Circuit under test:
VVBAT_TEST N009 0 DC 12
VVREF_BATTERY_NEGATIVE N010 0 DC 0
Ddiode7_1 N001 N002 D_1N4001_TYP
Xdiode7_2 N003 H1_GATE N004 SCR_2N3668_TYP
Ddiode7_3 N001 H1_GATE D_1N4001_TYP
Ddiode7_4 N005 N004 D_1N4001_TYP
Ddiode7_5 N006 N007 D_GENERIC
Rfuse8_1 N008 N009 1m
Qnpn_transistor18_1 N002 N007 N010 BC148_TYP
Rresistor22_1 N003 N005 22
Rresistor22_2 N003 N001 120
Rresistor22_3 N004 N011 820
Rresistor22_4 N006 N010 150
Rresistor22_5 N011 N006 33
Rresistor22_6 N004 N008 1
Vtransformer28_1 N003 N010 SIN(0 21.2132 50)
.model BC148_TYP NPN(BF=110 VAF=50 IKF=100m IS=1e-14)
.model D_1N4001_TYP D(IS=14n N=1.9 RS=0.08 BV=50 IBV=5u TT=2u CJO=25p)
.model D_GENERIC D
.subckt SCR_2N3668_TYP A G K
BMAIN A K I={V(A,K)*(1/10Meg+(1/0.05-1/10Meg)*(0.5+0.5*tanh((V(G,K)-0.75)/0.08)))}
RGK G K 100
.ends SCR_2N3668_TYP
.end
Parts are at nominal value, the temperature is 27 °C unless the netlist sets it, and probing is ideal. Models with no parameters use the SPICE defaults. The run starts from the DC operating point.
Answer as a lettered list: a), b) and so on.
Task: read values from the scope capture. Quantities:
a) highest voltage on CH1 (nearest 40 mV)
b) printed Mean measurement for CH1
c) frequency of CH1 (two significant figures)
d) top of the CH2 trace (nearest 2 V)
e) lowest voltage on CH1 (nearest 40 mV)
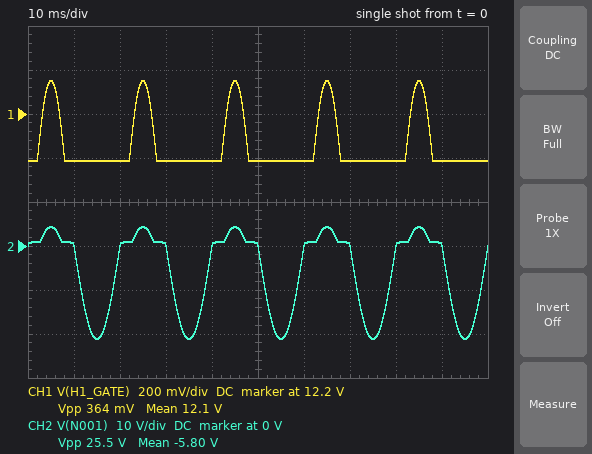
a) 12.36 V
b) 12.1 V
c) 50 Hz
d) 4 V
e) 12.00 V
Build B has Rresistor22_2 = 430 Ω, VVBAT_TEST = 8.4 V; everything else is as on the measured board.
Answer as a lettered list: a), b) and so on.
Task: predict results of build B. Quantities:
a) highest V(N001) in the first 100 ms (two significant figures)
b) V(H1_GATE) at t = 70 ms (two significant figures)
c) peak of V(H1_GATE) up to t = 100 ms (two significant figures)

a) 10 V
b) 8.4 V
c) 9.6 V
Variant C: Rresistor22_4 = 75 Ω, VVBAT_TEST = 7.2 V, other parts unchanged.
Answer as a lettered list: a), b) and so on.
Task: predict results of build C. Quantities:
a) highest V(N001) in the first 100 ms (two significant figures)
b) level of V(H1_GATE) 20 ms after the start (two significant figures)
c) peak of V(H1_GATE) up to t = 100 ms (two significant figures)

a) 18 V
b) 7.2 V
c) 17 V
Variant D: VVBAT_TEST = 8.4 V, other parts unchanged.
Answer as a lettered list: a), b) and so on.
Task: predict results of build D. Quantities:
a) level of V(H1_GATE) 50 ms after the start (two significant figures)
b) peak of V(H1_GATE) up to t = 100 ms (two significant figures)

a) 8.4 V
b) 11 V
